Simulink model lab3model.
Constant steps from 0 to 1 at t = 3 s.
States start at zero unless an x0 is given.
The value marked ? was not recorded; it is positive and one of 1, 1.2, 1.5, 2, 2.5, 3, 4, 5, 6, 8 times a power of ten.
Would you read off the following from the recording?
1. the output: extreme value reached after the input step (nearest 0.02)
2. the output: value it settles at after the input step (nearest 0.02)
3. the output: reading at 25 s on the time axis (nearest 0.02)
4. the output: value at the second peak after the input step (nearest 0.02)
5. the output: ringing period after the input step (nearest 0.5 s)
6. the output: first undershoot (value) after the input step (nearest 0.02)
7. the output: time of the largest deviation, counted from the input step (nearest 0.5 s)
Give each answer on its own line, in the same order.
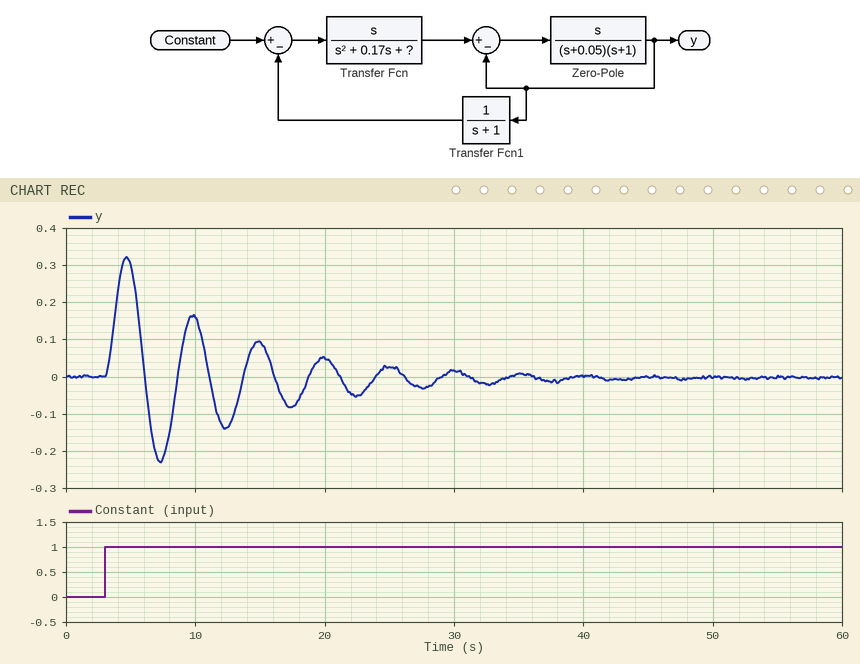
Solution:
0.32
0.00
0.02
0.16
5.0 s
-0.22
1.5 s
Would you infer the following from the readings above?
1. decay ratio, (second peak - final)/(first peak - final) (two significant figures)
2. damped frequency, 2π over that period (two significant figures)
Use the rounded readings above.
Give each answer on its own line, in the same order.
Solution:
0.50
1.3 rad/s
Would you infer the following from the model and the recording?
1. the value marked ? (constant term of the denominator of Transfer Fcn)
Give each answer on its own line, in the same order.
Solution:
1.2
